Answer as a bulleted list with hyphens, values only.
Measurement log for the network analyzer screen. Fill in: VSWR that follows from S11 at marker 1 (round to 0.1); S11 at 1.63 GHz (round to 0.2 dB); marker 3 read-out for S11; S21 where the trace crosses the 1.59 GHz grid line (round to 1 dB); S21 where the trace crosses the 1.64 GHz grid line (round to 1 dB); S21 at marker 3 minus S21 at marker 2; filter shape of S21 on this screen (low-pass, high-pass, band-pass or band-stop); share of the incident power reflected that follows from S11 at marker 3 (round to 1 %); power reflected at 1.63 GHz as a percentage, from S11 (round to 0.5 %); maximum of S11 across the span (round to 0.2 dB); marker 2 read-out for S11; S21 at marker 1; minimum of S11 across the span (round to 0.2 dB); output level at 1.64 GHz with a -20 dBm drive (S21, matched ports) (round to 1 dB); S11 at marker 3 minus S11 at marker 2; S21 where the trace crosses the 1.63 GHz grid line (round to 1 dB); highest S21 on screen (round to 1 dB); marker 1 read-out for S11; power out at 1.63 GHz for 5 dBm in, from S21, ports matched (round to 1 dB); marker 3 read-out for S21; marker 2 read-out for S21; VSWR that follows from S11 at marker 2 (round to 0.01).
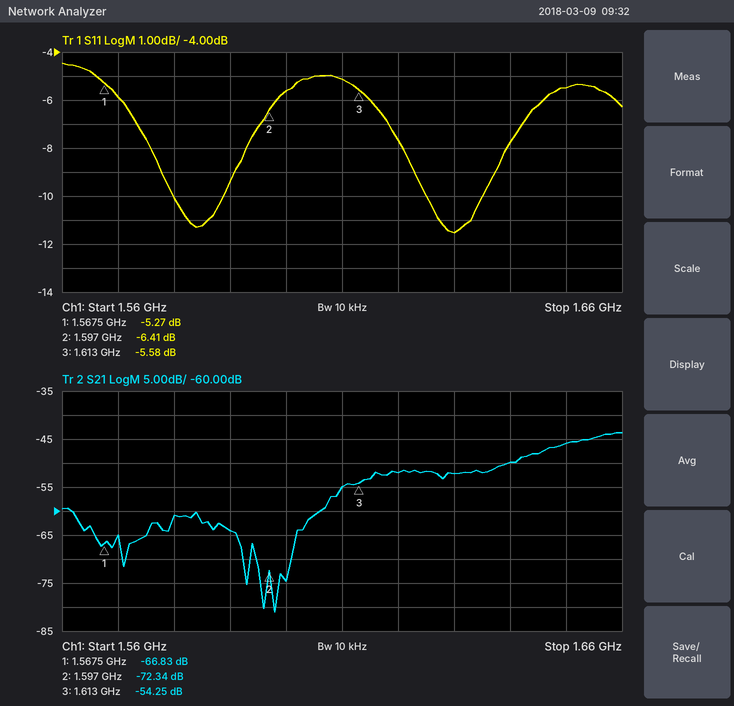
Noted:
- 3.4
- -11.6 dB
- -5.58 dB
- -64 dB
- -50 dB
- 18.09 dB
- high-pass
- 28 %
- 7.0 %
- -4.4 dB
- -6.41 dB
- -66.83 dB
- -11.6 dB
- -70 dBm
- 0.83 dB
- -52 dB
- -44 dB
- -5.27 dB
- -47 dBm
- -54.25 dB
- -72.34 dB
- 2.83
